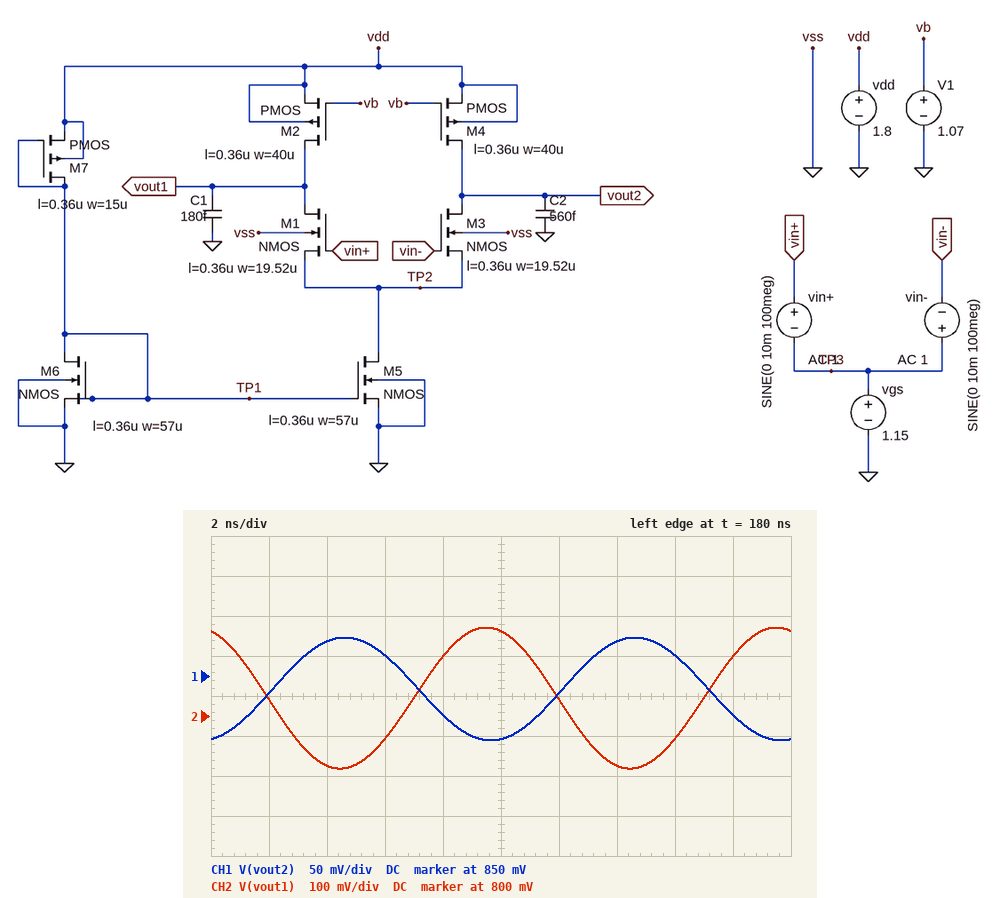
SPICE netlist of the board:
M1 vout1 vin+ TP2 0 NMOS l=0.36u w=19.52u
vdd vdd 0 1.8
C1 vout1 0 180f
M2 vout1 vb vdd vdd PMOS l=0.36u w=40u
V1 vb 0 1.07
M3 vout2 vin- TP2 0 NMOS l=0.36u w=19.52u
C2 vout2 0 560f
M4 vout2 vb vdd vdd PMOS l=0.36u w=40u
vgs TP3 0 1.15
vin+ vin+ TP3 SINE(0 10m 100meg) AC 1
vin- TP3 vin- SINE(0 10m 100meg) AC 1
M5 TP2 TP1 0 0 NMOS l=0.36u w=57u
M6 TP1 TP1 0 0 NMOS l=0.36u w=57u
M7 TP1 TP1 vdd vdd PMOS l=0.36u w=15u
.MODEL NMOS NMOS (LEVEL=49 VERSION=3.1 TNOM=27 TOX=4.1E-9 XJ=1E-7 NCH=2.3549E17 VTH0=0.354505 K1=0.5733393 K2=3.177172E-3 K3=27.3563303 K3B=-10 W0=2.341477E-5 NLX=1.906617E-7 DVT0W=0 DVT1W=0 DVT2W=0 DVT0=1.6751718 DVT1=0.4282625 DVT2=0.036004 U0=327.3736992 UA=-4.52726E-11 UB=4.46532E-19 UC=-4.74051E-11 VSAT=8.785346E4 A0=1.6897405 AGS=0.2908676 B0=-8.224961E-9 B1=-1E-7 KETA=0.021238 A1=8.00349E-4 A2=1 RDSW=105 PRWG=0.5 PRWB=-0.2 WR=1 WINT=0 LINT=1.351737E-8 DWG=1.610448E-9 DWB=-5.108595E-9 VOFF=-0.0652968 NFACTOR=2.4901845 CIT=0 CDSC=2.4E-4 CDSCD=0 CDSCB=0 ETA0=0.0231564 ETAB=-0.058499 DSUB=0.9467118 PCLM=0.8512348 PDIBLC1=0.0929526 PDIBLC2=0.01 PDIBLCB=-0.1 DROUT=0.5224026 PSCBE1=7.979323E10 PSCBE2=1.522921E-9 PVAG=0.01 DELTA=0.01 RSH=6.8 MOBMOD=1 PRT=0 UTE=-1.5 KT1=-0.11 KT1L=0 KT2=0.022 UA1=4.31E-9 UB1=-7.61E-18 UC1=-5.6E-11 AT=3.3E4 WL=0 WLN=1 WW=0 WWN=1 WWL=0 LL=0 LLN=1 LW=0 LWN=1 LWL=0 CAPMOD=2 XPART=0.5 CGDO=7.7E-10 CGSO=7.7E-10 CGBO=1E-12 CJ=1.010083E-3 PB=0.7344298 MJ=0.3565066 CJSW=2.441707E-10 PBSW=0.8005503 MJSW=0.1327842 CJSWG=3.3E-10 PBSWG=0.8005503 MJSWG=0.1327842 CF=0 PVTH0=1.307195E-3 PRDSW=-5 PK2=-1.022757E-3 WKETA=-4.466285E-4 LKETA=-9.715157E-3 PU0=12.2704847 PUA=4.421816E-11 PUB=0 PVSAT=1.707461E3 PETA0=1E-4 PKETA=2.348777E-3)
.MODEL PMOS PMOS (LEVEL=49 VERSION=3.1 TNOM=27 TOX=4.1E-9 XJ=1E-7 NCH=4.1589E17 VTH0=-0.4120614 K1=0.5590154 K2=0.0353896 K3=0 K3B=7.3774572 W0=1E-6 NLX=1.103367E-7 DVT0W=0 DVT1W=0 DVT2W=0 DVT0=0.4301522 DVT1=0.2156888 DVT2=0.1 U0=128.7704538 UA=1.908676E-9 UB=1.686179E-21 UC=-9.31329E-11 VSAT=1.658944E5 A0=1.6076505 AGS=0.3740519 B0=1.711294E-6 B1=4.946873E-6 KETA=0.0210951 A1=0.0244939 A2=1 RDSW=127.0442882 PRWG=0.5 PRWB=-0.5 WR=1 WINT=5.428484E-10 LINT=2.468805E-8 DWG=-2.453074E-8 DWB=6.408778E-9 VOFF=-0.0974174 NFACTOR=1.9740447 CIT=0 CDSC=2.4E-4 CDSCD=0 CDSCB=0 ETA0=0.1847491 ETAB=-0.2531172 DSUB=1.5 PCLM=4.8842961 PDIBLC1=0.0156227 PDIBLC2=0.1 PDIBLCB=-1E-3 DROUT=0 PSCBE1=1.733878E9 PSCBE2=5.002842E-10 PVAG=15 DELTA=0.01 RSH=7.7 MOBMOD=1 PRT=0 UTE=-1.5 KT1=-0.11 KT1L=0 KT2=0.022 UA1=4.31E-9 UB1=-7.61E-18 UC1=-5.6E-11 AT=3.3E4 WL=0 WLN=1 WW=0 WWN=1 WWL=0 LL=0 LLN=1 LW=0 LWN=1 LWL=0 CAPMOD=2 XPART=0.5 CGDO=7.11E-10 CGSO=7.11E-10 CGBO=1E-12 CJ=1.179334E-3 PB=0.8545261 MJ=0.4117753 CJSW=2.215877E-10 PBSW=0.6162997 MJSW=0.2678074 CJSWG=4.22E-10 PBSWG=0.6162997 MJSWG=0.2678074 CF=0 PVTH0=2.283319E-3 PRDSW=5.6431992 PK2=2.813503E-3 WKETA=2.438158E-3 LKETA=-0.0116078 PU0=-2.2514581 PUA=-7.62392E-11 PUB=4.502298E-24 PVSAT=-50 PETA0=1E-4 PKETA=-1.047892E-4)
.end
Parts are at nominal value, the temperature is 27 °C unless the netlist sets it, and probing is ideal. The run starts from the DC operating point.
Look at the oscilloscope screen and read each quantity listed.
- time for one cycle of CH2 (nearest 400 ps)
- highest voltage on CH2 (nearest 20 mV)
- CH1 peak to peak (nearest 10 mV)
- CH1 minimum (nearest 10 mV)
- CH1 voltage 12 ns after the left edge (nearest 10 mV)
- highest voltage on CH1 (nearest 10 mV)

10.0 ns
1.02 V
130 mV
770 mV
830 mV
900 mV
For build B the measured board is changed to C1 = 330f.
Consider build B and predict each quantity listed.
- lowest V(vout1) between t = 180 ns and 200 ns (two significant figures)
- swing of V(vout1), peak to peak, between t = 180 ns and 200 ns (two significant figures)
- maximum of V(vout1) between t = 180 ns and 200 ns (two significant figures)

730 mV
220 mV
950 mV
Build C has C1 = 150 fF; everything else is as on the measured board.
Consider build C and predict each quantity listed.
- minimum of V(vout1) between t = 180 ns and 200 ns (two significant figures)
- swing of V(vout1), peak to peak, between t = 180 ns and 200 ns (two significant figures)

650 mV
400 mV
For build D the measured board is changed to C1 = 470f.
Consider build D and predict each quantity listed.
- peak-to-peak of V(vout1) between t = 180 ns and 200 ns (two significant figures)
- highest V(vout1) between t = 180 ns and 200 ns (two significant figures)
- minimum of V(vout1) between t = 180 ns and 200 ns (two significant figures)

160 mV
920 mV
760 mV
